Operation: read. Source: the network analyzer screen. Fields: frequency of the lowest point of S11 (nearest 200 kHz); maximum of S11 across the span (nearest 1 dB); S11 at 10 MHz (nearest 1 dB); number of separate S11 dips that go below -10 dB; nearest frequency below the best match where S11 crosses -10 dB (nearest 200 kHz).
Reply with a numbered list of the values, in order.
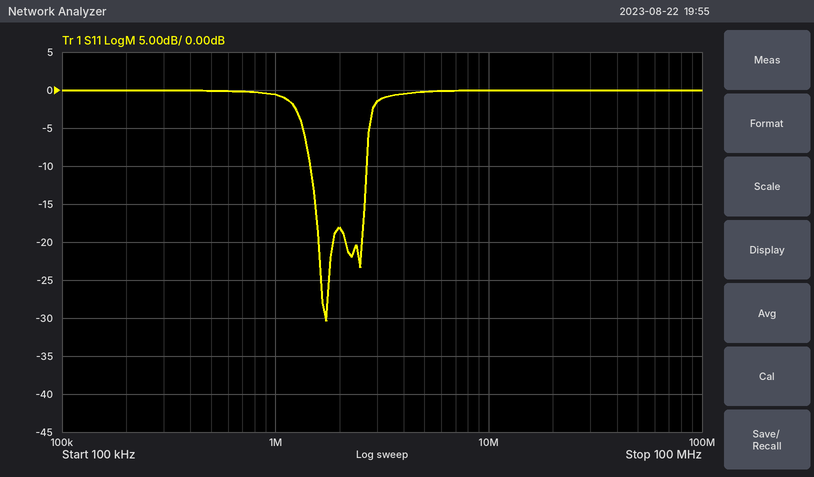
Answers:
1. 1.8 MHz
2. 0 dB
3. 0 dB
4. 2
5. 1.4 MHz
